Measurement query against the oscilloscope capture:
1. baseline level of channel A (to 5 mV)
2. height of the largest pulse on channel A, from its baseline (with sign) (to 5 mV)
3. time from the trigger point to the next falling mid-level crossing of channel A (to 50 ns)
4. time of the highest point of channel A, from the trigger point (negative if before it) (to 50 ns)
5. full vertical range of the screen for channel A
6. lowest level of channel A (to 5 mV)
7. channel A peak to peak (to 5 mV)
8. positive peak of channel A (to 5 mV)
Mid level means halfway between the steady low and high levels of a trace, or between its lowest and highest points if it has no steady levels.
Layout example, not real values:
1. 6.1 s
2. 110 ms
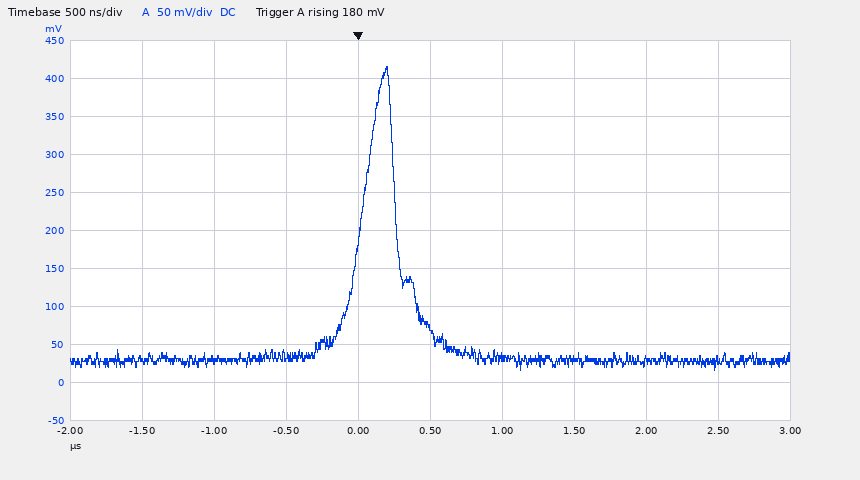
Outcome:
1. 30 mV
2. +385 mV
3. 250 ns
4. +200 ns
5. 500 mV
6. 15 mV
7. 400 mV
8. 415 mV
